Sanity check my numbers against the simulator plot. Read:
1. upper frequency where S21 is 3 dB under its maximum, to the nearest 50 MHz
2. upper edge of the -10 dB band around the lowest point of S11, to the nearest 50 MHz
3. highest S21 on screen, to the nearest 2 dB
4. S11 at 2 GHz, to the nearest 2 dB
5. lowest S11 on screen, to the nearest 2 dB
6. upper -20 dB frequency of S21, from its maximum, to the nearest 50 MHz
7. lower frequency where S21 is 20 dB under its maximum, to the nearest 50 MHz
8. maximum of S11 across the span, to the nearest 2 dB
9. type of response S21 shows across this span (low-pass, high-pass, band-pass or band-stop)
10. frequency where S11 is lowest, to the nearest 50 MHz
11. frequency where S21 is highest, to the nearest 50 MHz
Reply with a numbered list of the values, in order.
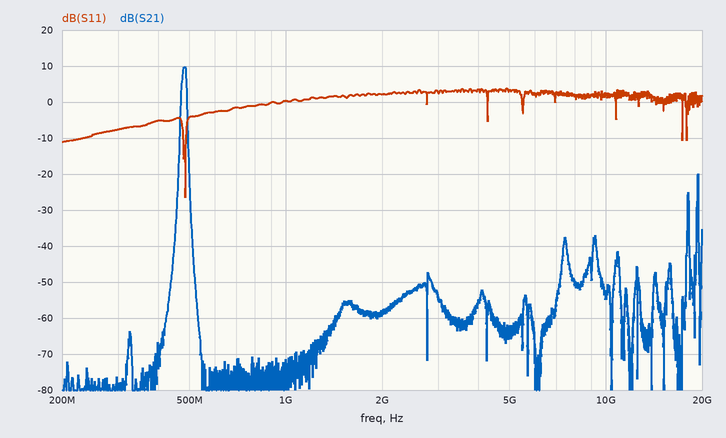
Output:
1. 500 MHz
2. 500 MHz
3. 10 dB
4. 2 dB
5. -26 dB
6. 500 MHz
7. 450 MHz
8. 4 dB
9. band-pass
10. 500 MHz
11. 500 MHz
